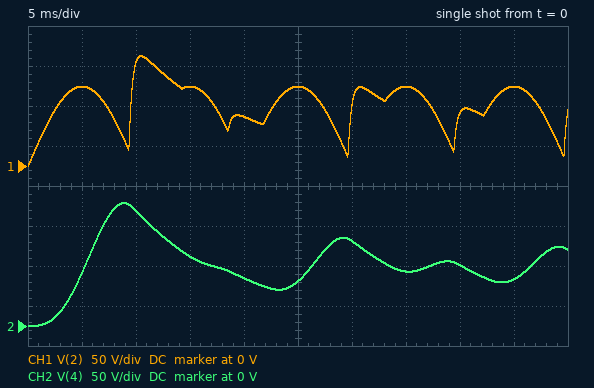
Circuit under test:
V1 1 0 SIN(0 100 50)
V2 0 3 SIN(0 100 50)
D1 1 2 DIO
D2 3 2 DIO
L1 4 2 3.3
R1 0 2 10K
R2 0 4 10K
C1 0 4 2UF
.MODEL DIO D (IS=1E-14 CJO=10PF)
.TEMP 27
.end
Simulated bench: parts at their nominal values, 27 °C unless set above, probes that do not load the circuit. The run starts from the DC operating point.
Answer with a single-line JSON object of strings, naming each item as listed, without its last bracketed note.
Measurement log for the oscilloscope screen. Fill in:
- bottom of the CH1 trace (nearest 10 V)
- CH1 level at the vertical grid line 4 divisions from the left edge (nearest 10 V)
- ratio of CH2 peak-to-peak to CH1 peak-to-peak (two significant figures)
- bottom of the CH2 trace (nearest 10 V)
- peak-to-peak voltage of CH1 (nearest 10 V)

{"bottom of the CH1 trace": "0 V", "CH1 level at the vertical grid line 4 divisions from the left edge": "60 V", "ratio of CH2 peak-to-peak to CH1 peak-to-peak": "1.1", "bottom of the CH2 trace": "0 V", "peak-to-peak voltage of CH1": "140 V"}
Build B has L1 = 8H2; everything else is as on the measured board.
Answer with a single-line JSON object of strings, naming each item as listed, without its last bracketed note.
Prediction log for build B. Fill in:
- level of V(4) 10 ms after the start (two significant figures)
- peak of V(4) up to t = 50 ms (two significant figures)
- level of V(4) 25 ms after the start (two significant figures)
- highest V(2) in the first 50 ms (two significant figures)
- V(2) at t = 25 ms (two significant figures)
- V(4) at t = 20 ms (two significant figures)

{"level of V(4) 10 ms after the start": "110 V", "peak of V(4) up to t = 50 ms": "120 V", "level of V(4) 25 ms after the start": "47 V", "highest V(2) in the first 50 ms": "99 V", "V(2) at t = 25 ms": "99 V", "V(4) at t = 20 ms": "68 V"}
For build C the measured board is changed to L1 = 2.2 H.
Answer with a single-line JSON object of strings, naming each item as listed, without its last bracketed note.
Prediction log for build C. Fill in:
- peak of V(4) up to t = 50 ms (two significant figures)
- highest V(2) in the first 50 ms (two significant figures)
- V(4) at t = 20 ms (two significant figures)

{"peak of V(4) up to t = 50 ms": "160 V", "highest V(2) in the first 50 ms": "150 V", "V(4) at t = 20 ms": "66 V"}
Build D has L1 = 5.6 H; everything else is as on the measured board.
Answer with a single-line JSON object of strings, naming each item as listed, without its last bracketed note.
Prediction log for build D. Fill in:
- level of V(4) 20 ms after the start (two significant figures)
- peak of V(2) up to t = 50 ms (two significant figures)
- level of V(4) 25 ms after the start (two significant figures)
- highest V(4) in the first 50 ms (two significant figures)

{"level of V(4) 20 ms after the start": "56 V", "peak of V(2) up to t = 50 ms": "110 V", "level of V(4) 25 ms after the start": "46 V", "highest V(4) in the first 50 ms": "130 V"}
